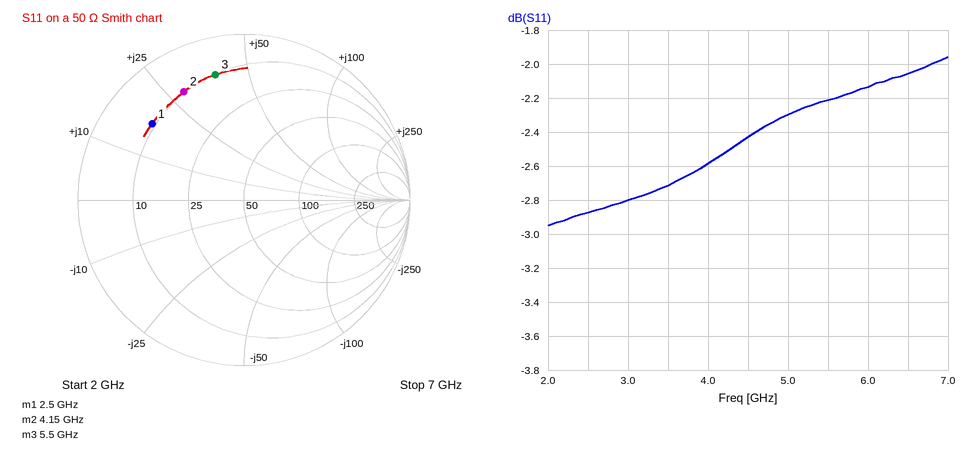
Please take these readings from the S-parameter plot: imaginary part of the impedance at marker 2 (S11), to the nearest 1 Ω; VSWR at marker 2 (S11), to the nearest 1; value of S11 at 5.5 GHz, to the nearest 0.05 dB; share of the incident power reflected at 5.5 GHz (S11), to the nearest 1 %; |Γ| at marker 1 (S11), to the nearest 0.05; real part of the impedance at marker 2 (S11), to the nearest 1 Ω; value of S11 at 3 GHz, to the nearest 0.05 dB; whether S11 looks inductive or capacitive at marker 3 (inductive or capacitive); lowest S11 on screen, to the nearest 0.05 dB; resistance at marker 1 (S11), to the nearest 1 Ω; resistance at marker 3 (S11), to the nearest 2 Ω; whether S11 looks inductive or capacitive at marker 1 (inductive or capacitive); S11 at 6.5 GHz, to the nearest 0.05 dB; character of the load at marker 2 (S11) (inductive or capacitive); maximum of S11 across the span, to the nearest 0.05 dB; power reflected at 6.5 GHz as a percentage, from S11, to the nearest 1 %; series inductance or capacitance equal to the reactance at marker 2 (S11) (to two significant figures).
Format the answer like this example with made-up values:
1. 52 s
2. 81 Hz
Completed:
1. +29 Ω
2. 7
3. -2.20 dB
4. 60 %
5. 0.70
6. 10 Ω
7. -2.80 dB
8. inductive
9. -2.95 dB
10. 9 Ω
11. 10 Ω
12. inductive
13. -2.05 dB
14. inductive
15. -1.95 dB
16. 62 %
17. 1.1 nH
